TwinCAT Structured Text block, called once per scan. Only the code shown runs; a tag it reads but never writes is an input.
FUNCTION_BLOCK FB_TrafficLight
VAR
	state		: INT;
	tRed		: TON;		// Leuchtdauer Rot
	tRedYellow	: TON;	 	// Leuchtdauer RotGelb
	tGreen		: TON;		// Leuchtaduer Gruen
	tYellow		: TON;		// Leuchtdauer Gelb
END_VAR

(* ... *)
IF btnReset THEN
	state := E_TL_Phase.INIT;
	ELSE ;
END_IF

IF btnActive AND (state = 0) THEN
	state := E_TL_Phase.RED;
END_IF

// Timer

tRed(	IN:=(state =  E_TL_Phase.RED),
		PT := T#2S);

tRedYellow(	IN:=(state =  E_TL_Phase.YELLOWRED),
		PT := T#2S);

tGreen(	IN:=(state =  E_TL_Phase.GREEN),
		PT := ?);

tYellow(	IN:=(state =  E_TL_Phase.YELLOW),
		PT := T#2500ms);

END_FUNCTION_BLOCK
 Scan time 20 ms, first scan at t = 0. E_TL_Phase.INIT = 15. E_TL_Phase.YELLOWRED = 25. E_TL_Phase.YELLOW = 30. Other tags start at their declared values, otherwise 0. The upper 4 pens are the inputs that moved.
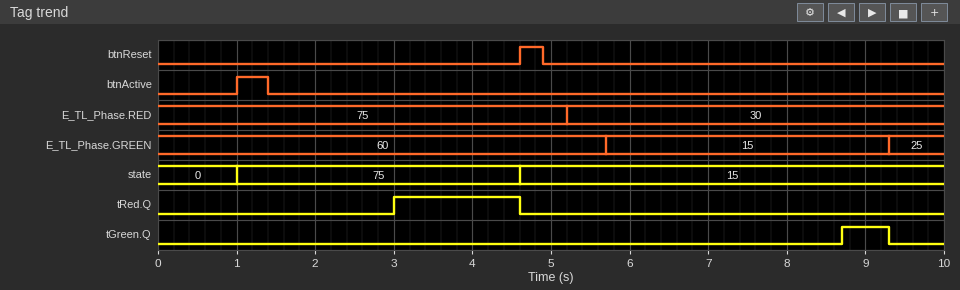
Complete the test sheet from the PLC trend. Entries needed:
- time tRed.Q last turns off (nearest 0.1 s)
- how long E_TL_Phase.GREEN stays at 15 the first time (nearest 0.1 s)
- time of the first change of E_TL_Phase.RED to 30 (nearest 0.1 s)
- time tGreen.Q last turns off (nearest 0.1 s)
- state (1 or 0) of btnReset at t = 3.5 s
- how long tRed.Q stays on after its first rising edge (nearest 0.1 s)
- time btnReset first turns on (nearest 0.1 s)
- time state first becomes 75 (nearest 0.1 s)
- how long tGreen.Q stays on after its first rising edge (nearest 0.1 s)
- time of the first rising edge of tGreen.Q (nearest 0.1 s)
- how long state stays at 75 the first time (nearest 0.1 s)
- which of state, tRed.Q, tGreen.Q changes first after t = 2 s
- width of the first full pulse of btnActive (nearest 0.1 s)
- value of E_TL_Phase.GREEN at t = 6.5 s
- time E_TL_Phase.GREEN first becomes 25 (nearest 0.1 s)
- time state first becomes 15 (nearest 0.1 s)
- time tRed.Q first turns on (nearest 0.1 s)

4.6 s
3.6 s
5.2 s
9.3 s
0
1.6 s
4.6 s
1.0 s
0.6 s
8.7 s
3.6 s
tRed.Q
0.4 s
15
9.3 s
4.6 s
3.0 s
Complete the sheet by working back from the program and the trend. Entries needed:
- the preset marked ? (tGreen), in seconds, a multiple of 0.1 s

3.0 s
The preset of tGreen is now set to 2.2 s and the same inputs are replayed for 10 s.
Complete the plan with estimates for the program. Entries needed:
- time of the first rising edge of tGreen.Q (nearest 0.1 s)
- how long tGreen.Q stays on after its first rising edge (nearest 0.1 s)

7.9 s
1.4 s
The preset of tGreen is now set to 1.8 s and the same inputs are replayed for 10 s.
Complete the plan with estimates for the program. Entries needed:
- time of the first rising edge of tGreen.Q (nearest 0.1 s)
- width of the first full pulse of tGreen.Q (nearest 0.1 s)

7.5 s
1.8 s
